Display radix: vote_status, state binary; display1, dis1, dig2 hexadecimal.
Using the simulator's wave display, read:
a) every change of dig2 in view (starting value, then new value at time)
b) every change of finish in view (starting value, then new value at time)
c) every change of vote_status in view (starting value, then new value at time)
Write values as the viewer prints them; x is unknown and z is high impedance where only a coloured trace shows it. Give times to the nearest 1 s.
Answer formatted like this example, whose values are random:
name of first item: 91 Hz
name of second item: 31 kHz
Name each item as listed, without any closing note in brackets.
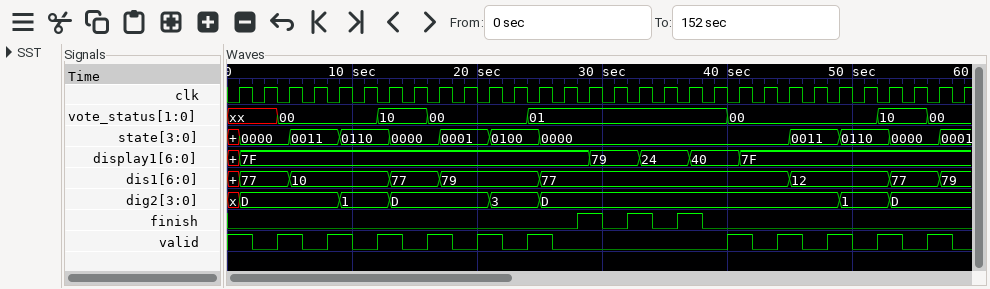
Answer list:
every change of dig2 in view: x, D at 1 s, 1 at 9 s, D at 13 s, 3 at 21 s, D at 25 s, 1 at 49 s, D at 53 s
every change of finish in view: 0, 1 at 28 s, 0 at 30 s, 1 at 32 s, 0 at 34 s, 1 at 36 s, 0 at 38 s
every change of vote_status in view: xx, 00 at 4 s, 10 at 12 s, 00 at 16 s, 01 at 24 s, 00 at 40 s, 10 at 52 s, 00 at 56 s
